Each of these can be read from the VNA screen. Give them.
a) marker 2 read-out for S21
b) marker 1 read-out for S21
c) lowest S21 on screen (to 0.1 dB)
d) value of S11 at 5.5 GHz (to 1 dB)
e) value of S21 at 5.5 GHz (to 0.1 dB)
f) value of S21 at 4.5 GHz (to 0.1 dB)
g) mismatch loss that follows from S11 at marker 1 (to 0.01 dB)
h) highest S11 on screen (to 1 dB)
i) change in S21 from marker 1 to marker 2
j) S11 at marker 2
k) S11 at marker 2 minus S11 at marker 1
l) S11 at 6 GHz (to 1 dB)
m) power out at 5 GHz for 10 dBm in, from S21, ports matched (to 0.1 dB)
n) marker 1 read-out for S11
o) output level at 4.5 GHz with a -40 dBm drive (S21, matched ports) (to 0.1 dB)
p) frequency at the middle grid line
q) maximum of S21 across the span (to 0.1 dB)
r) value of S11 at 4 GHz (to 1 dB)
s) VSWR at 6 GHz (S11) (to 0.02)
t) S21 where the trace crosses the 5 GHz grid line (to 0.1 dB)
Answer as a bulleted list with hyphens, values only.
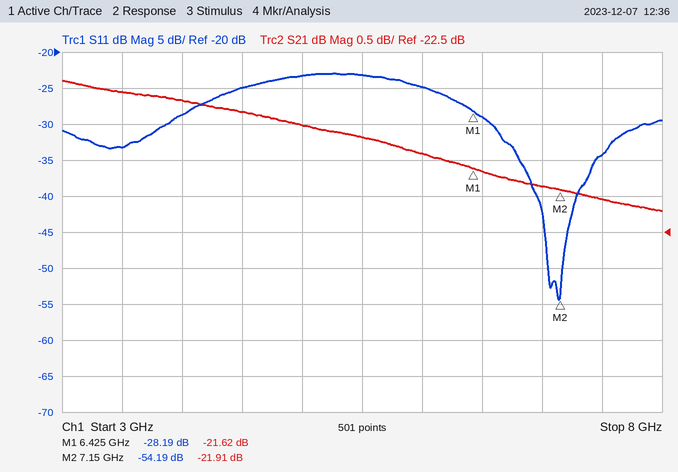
- -21.91 dB
- -21.62 dB
- -22.2 dB
- -23 dB
- -21.2 dB
- -20.8 dB
- 0.01 dB
- -23 dB
- -0.29 dB
- -54.19 dB
- -26.00 dB
- -25 dB
- -11.0 dBm
- -28.19 dB
- -60.8 dBm
- 5.5 GHz
- -20.4 dB
- -29 dB
- 1.12
- -21.0 dB
